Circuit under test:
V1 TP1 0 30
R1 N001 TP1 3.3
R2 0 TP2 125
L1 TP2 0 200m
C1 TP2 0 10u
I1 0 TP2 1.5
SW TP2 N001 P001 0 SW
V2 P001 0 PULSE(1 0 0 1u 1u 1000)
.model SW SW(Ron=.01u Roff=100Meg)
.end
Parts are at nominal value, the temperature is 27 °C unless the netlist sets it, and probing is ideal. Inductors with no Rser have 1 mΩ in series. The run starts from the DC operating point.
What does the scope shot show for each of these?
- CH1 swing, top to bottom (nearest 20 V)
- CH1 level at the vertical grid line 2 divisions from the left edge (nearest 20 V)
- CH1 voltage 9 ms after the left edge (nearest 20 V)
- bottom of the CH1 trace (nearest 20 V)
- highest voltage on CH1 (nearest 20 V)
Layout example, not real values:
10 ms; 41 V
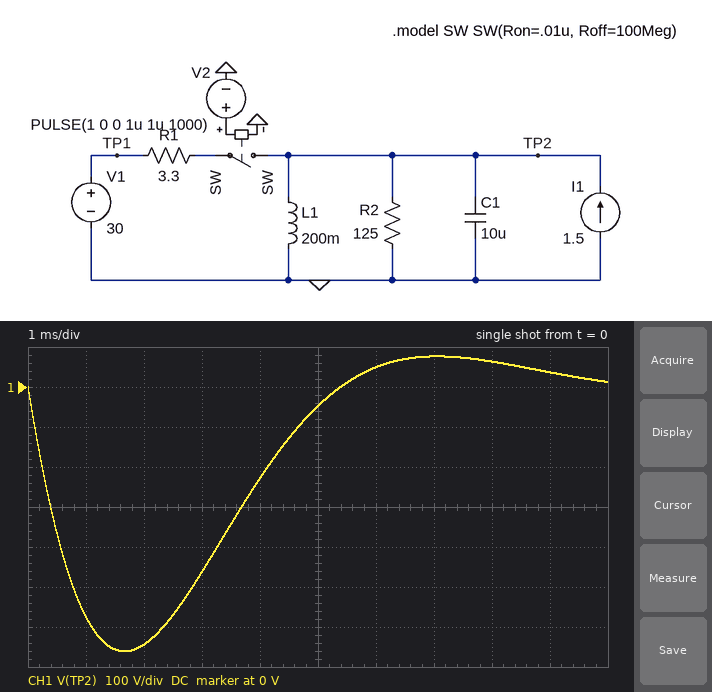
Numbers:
740 V; -640 V; 40 V; -660 V; 80 V
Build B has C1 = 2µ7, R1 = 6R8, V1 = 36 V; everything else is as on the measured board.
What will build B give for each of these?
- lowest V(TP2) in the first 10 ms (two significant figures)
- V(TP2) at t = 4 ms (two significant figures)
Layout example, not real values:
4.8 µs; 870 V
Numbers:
-500 V; -46 V
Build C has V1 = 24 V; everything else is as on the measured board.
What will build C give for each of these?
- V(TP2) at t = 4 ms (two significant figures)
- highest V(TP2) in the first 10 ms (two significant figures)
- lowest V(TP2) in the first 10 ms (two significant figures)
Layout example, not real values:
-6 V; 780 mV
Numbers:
-180 V; 61 V; -530 V
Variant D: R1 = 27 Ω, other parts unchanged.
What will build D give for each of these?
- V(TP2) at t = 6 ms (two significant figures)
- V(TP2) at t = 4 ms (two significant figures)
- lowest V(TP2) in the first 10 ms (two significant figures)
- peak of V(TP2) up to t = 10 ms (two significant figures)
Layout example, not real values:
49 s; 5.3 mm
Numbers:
6.0 V; -28 V; -81 V; 9.4 V
